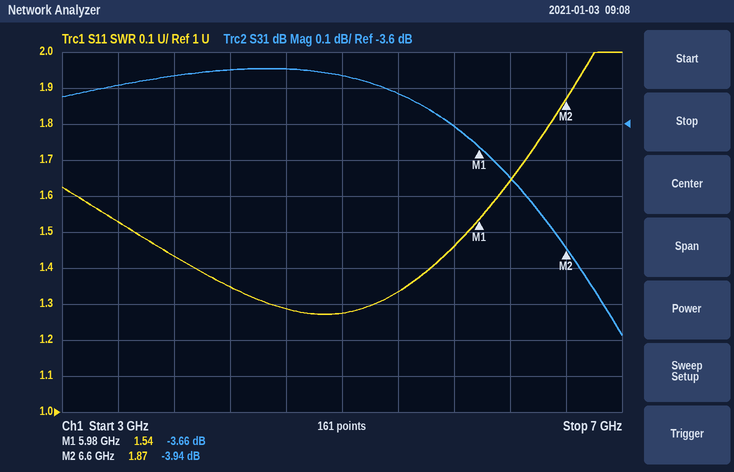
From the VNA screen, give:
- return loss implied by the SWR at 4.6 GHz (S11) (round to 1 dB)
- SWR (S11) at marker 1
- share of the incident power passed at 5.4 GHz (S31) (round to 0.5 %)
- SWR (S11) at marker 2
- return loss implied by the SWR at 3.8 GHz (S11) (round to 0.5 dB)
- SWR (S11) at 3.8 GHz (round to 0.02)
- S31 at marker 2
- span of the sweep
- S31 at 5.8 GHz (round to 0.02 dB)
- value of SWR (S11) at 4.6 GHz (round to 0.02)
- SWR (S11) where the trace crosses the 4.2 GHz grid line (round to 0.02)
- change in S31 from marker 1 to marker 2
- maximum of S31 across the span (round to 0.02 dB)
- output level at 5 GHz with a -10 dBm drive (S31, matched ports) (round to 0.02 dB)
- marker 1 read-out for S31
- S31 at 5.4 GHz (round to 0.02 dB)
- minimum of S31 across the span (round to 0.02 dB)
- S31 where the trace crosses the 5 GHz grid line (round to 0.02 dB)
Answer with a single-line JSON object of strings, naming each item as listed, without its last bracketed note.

{"return loss implied by the SWR at 4.6 GHz (S11)": "18 dB", "SWR (S11) at marker 1": "1.54", "share of the incident power passed at 5.4 GHz (S31)": "44.5 %", "SWR (S11) at marker 2": "1.87", "return loss implied by the SWR at 3.8 GHz (S11)": "15.0 dB", "SWR (S11) at 3.8 GHz": "1.44", "S31 at marker 2": "-3.94 dB", "span of the sweep": "4 GHz", "S31 at 5.8 GHz": "-3.60 dB", "value of SWR (S11) at 4.6 GHz": "1.28", "SWR (S11) where the trace crosses the 4.2 GHz grid line": "1.34", "change in S31 from marker 1 to marker 2": "-0.28 dB", "maximum of S31 across the span": "-3.44 dB", "output level at 5 GHz with a -10 dBm drive (S31, matched ports)": "-13.46 dBm", "marker 1 read-out for S31": "-3.66 dB", "S31 at 5.4 GHz": "-3.52 dB", "minimum of S31 across the span": "-4.18 dB", "S31 where the trace crosses the 5 GHz grid line": "-3.46 dB"}
